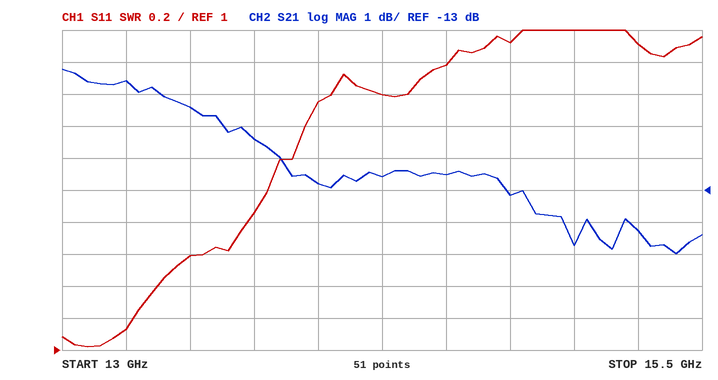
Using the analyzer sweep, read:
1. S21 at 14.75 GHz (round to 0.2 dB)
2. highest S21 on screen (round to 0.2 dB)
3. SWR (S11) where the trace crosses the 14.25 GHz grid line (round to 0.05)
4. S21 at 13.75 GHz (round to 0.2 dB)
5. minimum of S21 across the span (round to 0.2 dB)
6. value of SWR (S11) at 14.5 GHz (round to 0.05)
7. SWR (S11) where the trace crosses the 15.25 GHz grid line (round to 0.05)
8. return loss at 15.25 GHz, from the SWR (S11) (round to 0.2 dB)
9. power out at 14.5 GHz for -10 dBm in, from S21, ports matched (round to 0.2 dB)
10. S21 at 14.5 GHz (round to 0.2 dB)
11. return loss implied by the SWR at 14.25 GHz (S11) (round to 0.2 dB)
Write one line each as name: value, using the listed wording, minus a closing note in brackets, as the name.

S21 at 14.75 GHz: -13.2 dB
highest S21 on screen: -9.2 dB
SWR (S11) where the trace crosses the 14.25 GHz grid line: 2.60
S21 at 13.75 GHz: -11.4 dB
minimum of S21 across the span: -15.0 dB
value of SWR (S11) at 14.5 GHz: 2.80
SWR (S11) where the trace crosses the 15.25 GHz grid line: 2.90
return loss at 15.25 GHz, from the SWR (S11): 6.2 dB
power out at 14.5 GHz for -10 dBm in, from S21, ports matched: -22.6 dBm
S21 at 14.5 GHz: -12.6 dB
return loss implied by the SWR at 14.25 GHz (S11): 7.0 dB
